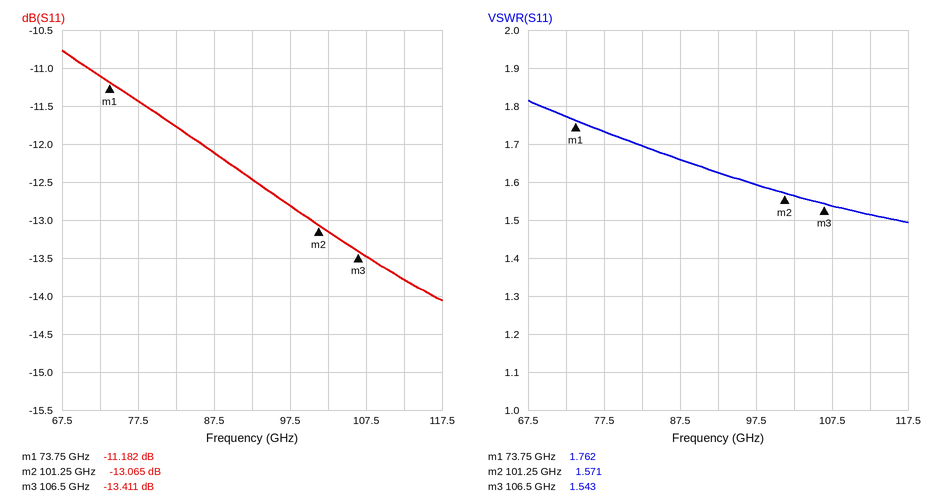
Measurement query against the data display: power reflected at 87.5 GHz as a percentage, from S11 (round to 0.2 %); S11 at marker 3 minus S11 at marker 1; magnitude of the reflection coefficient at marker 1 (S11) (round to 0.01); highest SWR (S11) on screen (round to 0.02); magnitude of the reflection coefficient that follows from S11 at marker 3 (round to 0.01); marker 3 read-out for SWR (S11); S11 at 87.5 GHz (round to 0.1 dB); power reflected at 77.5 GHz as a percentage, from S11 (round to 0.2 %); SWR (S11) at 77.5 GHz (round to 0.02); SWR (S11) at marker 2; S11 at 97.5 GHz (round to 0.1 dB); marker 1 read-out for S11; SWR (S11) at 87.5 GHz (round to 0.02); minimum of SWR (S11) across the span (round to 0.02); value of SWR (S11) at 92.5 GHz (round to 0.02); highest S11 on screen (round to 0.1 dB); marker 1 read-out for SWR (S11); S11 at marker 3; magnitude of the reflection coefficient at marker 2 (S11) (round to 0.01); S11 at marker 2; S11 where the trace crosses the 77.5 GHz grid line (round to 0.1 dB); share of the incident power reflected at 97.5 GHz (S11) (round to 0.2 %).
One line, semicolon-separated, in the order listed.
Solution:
6.2 %; -2.229 dB; 0.28; 1.82; 0.21; 1.543; -12.1 dB; 7.2 %; 1.74; 1.571; -12.8 dB; -11.182 dB; 1.66; 1.50; 1.62; -10.8 dB; 1.762; -13.411 dB; 0.22; -13.065 dB; -11.4 dB; 5.2 %
